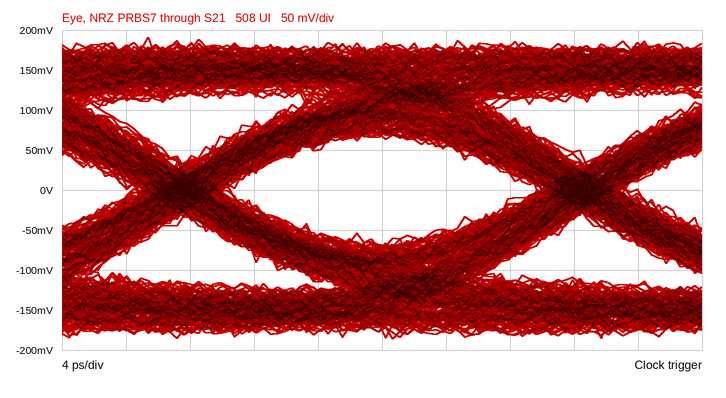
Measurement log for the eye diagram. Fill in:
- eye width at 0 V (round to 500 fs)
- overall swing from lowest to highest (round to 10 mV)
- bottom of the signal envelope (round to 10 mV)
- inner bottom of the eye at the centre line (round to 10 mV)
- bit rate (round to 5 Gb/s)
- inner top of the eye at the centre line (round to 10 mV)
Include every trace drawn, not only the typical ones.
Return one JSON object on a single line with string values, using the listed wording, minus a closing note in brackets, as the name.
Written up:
{"eye width at 0 V": "19.0 ps", "overall swing from lowest to highest": "380 mV", "bottom of the signal envelope": "-190 mV", "inner bottom of the eye at the centre line": "-70 mV", "bit rate": "40 Gb/s", "inner top of the eye at the centre line": "70 mV"}
